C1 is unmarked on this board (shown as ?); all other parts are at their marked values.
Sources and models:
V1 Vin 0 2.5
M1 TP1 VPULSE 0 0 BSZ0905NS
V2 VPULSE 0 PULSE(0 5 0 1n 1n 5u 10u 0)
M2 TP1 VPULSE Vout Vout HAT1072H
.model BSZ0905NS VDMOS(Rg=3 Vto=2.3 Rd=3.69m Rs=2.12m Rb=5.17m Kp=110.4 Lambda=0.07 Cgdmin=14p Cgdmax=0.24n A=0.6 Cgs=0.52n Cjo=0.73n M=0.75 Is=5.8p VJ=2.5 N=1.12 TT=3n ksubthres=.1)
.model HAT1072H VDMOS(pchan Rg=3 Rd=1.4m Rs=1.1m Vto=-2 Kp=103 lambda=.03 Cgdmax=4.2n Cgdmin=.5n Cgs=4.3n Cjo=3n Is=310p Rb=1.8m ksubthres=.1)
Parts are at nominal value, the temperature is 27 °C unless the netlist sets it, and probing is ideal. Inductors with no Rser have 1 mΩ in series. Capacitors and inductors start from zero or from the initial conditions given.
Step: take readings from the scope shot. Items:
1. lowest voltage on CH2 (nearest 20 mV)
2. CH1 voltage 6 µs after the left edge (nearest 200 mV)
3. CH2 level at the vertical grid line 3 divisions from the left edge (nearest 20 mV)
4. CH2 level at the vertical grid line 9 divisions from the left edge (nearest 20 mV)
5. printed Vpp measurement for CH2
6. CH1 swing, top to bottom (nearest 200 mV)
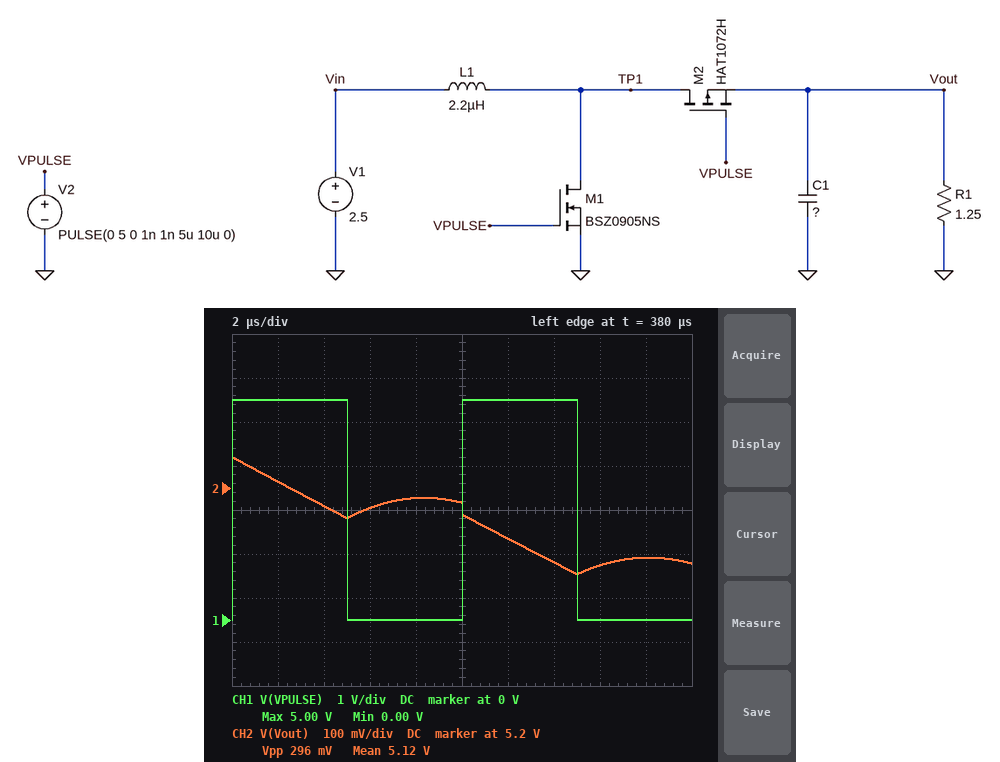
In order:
5.00 V
0 V
5.16 V
5.04 V
296 mV
5.0 V
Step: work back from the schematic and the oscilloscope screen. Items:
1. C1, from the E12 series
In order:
150 µF
